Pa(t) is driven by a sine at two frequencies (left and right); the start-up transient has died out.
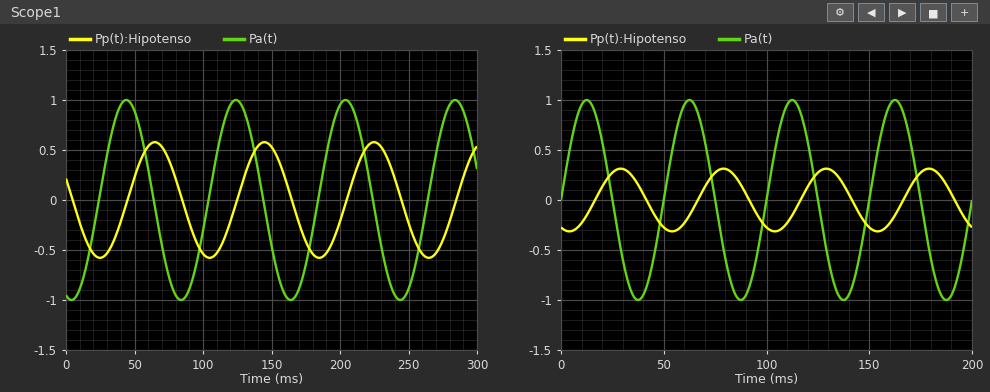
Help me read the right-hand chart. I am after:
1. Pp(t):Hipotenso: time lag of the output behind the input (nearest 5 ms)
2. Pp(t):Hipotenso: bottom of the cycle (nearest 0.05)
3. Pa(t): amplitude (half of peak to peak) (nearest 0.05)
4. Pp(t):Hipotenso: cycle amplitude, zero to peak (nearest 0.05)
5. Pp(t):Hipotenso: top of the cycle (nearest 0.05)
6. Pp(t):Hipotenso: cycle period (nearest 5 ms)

15 ms
-0.30
1.00
0.30
0.30
50 ms
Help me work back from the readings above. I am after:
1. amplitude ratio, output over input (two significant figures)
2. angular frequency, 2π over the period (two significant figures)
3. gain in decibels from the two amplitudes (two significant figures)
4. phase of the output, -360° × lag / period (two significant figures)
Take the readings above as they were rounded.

0.30
0.13 rad/ms
-10 dB
-110°
